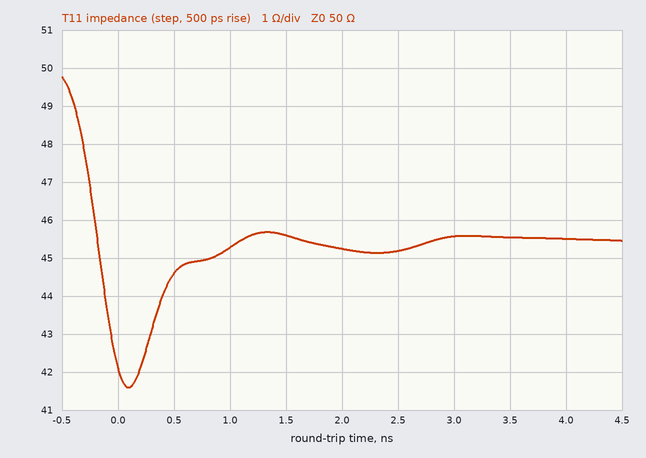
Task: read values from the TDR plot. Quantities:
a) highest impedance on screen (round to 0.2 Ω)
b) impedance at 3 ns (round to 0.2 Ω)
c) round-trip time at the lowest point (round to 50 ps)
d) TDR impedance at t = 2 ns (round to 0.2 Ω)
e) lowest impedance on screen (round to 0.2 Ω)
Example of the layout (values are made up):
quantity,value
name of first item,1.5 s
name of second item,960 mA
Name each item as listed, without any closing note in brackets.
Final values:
quantity,value
highest impedance on screen,49.8 Ω
impedance at 3 ns,45.6 Ω
round-trip time at the lowest point,100 ps
TDR impedance at t = 2 ns,45.2 Ω
lowest impedance on screen,41.6 Ω
